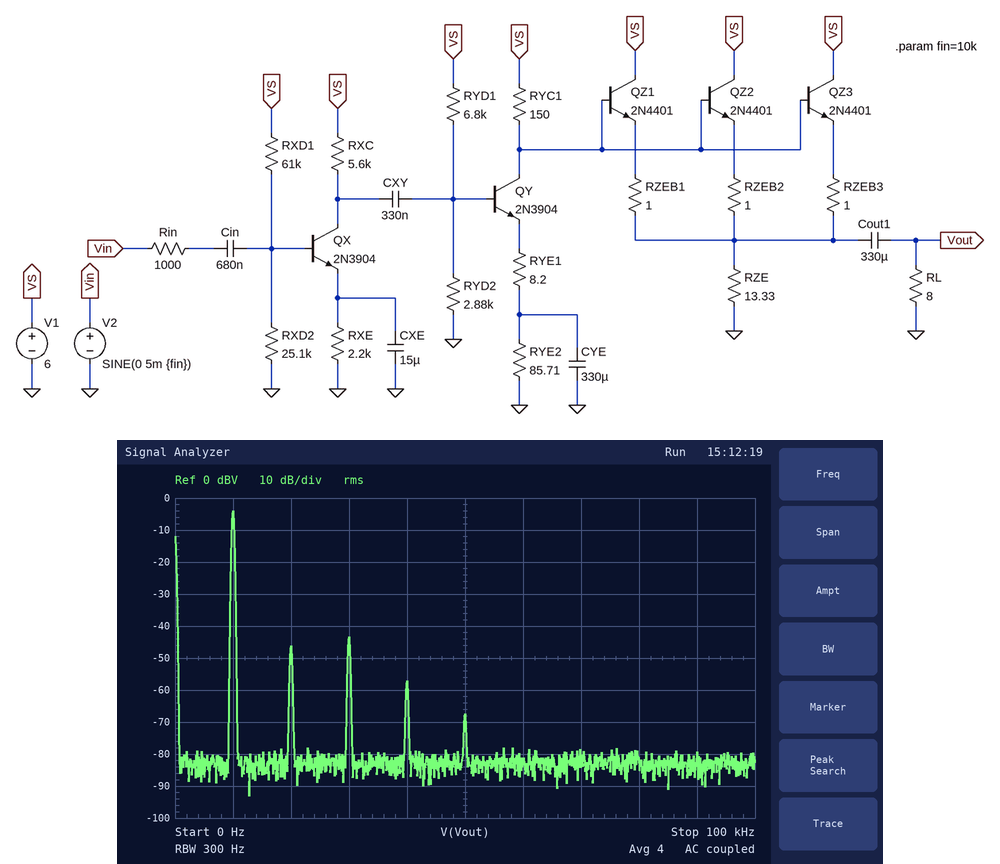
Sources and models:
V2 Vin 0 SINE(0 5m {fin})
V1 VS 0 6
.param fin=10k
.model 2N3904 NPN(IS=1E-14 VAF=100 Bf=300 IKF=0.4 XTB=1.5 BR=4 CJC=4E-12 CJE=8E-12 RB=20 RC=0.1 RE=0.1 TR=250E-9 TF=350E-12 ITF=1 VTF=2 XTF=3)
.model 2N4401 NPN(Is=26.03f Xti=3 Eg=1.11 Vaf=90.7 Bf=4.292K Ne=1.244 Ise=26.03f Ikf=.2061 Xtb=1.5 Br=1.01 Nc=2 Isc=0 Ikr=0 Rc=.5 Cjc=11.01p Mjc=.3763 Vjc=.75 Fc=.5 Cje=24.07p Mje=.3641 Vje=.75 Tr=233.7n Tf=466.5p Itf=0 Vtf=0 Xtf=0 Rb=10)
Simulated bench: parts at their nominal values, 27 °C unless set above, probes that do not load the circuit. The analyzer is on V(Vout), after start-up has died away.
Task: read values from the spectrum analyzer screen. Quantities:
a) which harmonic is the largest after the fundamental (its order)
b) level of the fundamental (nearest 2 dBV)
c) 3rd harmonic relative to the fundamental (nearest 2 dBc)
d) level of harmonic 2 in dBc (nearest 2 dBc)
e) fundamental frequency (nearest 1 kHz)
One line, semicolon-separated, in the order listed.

3; -4 dBV; -40 dBc; -42 dBc; 10 kHz
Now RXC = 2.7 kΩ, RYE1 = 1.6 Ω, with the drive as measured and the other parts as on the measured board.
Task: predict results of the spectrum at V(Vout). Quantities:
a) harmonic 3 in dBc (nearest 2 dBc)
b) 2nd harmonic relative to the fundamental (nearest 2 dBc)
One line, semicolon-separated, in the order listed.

-28 dBc; -28 dBc
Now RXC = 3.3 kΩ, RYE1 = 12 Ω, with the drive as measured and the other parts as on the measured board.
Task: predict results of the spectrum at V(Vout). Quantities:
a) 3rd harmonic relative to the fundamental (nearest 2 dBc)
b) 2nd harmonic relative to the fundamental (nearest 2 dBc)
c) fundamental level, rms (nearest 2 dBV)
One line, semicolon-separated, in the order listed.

-48 dBc; -34 dBc; -6 dBV
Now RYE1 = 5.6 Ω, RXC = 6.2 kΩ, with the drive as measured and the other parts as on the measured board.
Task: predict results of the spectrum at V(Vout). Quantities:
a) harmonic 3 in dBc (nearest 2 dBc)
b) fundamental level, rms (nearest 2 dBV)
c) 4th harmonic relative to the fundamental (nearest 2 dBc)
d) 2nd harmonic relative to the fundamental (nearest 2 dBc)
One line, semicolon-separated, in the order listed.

-34 dBc; -2 dBV; -50 dBc; -44 dBc
